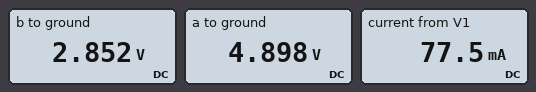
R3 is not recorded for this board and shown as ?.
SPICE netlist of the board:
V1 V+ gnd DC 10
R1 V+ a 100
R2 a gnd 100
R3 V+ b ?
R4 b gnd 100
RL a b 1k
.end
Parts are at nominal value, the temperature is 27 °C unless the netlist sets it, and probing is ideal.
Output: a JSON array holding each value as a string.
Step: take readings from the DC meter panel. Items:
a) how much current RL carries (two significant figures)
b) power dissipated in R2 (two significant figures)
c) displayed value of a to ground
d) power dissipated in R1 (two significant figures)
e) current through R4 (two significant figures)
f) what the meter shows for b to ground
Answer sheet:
["2.0 mA", "240 mW", "4.898 V", "260 mW", "29 mA", "2.852 V"]
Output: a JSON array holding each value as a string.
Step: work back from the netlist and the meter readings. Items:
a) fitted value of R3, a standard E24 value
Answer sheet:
["270 Ω"]
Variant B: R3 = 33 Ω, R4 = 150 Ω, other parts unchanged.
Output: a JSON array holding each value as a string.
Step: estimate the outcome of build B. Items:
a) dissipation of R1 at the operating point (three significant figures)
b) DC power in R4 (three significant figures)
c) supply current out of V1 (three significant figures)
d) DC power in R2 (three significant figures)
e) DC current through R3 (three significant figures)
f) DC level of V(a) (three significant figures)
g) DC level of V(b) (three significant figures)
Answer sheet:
["235 mW", "439 mW", "106 mA", "265 mW", "57.1 mA", "5.15 V", "8.12 V"]
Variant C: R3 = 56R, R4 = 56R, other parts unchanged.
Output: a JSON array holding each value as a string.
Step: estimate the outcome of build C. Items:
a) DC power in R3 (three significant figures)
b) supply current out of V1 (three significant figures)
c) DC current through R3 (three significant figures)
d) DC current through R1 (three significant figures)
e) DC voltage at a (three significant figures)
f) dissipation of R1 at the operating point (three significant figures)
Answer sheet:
["446 mW", "139 mA", "89.3 mA", "50.0 mA", "5.00 V", "250 mW"]
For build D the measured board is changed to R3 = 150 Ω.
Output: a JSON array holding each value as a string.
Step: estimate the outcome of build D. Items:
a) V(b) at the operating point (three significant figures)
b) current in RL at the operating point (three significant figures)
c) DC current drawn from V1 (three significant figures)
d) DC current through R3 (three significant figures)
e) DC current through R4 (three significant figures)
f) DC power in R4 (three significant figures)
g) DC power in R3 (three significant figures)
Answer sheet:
["4.05 V", "901 µA", "90.1 mA", "39.6 mA", "40.5 mA", "164 mW", "236 mW"]
